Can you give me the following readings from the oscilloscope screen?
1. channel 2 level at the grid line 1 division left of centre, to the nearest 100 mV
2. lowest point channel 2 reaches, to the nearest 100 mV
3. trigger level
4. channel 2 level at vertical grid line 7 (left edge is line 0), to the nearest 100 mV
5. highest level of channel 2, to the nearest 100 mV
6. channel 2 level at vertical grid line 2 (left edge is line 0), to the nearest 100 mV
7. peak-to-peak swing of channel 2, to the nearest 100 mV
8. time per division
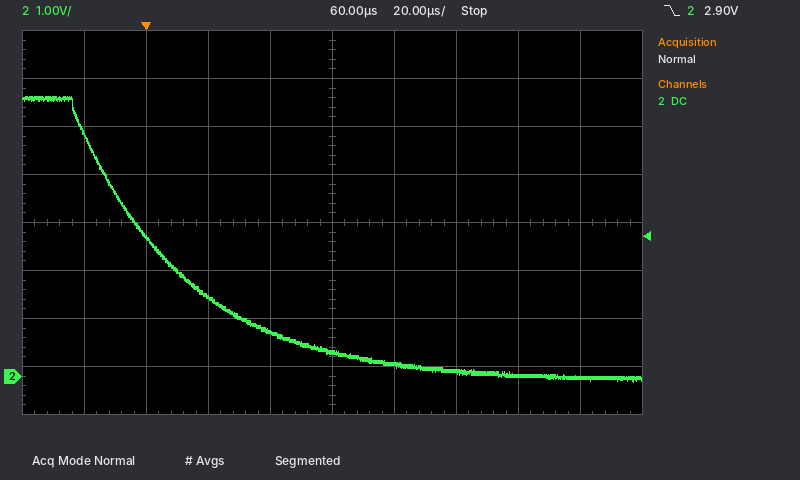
900 mV
-100 mV
2.90 V
100 mV
5.8 V
2.9 V
5.9 V
20 µs
